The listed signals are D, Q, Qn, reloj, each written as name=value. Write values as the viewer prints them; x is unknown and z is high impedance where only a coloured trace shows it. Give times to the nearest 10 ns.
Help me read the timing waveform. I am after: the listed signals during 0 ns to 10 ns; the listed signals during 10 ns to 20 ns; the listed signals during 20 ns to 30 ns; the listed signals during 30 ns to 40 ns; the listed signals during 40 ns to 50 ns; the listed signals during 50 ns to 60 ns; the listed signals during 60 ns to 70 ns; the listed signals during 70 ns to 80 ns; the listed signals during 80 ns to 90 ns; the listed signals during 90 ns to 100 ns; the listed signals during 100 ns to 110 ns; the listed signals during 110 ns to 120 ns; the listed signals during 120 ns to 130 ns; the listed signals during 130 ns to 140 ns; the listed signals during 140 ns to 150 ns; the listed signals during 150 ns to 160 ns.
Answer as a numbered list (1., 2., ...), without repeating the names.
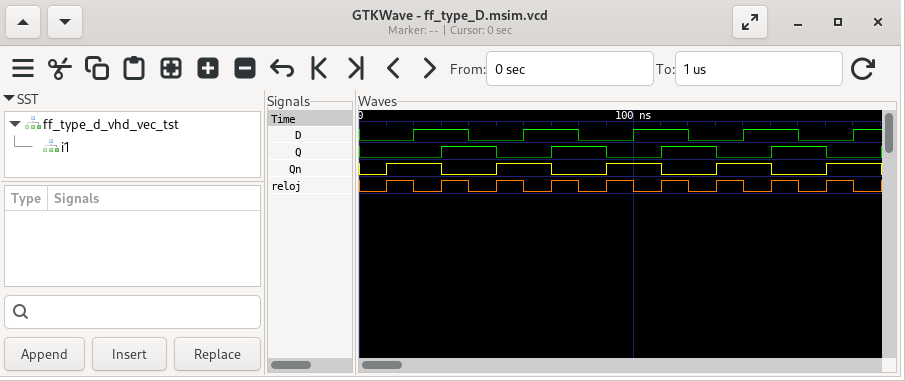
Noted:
1. D=0, Q=0, Qn=0, reloj=0
2. D=0, Q=0, Qn=1, reloj=1
3. D=1, Q=0, Qn=1, reloj=0
4. D=1, Q=1, Qn=0, reloj=1
5. D=0, Q=1, Qn=0, reloj=0
6. D=0, Q=0, Qn=1, reloj=1
7. D=1, Q=0, Qn=1, reloj=0
8. D=1, Q=1, Qn=0, reloj=1
9. D=0, Q=1, Qn=0, reloj=0
10. D=0, Q=0, Qn=1, reloj=1
11. D=1, Q=0, Qn=1, reloj=0
12. D=1, Q=1, Qn=0, reloj=1
13. D=0, Q=1, Qn=0, reloj=0
14. D=0, Q=0, Qn=1, reloj=1
15. D=1, Q=0, Qn=1, reloj=0
16. D=1, Q=1, Qn=0, reloj=1
